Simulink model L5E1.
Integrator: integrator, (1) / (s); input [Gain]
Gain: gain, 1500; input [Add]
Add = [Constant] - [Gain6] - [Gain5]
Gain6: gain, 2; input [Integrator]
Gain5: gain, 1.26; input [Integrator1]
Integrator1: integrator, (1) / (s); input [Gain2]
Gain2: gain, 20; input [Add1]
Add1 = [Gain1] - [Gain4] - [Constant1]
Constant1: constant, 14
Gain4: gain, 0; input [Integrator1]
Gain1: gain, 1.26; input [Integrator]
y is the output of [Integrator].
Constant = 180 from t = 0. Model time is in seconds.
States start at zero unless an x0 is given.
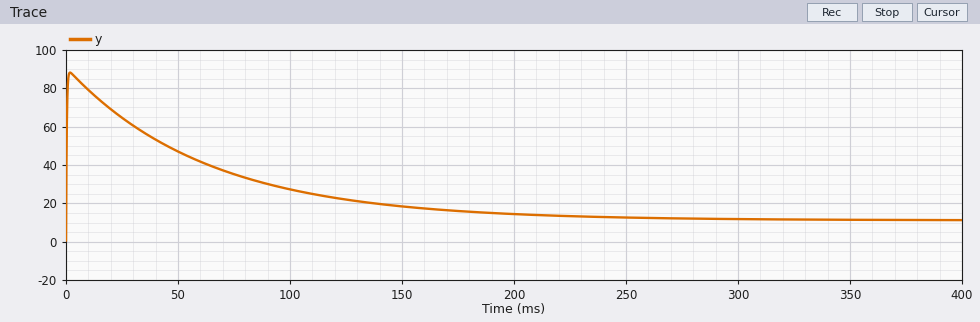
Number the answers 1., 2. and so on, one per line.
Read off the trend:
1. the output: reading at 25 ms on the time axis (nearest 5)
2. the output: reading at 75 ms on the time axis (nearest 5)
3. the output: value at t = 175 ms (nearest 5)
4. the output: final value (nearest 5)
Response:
1. 65
2. 35
3. 15
4. 10
